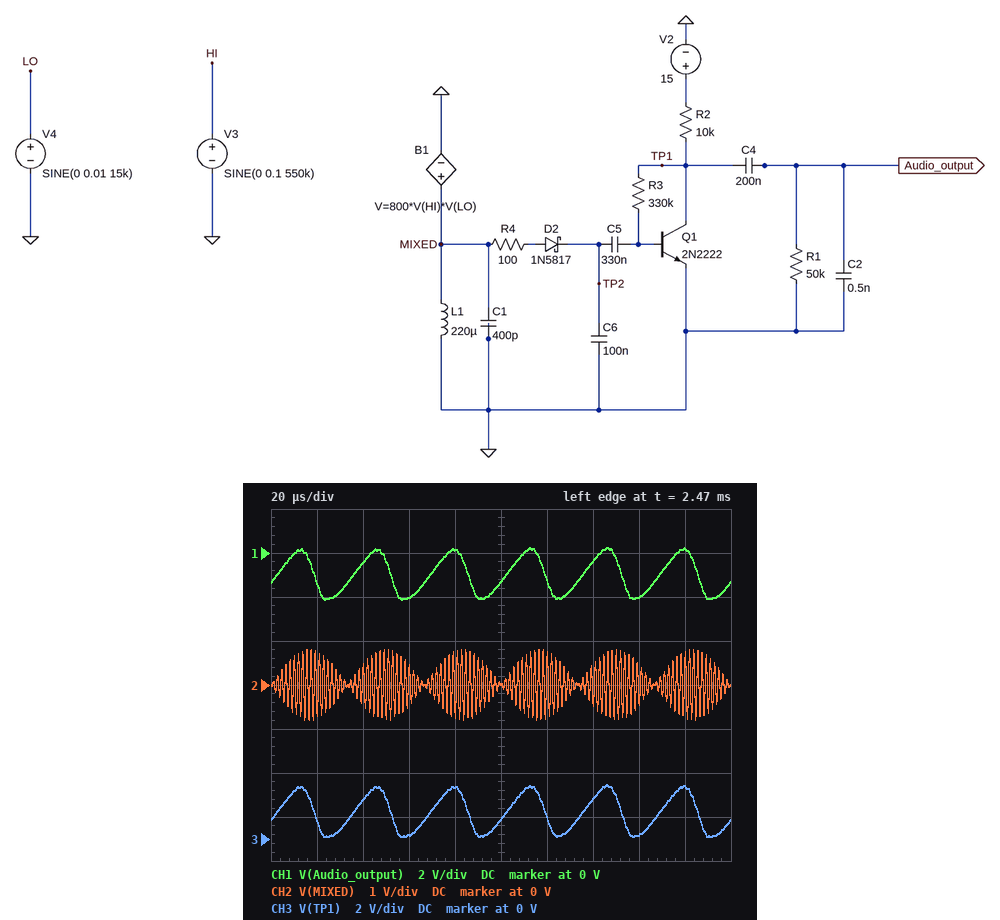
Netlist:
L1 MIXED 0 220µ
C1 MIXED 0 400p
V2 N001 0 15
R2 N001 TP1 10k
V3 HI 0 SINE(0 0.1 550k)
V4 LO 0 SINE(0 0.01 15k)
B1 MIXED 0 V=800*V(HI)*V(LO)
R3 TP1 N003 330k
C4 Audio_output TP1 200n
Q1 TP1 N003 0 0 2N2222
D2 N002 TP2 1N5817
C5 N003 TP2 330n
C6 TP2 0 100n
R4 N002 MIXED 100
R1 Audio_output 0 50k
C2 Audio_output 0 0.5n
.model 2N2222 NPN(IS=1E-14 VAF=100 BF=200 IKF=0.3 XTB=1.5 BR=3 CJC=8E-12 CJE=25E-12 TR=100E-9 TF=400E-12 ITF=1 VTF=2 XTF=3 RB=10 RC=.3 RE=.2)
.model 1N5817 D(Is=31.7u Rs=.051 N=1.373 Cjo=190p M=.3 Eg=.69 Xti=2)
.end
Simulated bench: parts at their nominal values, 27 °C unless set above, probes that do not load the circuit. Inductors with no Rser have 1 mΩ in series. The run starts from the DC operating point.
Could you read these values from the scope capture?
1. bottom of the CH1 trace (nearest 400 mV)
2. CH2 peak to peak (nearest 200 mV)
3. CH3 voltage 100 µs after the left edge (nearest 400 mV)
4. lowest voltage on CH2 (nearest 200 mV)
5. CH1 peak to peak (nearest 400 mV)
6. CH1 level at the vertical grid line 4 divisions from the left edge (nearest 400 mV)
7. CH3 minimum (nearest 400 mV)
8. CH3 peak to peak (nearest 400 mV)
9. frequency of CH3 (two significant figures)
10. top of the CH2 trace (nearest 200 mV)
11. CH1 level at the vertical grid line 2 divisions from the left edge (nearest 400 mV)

-2.0 V
1.6 V
800 mV
-800 mV
2.4 V
0 V
0 V
2.4 V
30 kHz
800 mV
-400 mV
